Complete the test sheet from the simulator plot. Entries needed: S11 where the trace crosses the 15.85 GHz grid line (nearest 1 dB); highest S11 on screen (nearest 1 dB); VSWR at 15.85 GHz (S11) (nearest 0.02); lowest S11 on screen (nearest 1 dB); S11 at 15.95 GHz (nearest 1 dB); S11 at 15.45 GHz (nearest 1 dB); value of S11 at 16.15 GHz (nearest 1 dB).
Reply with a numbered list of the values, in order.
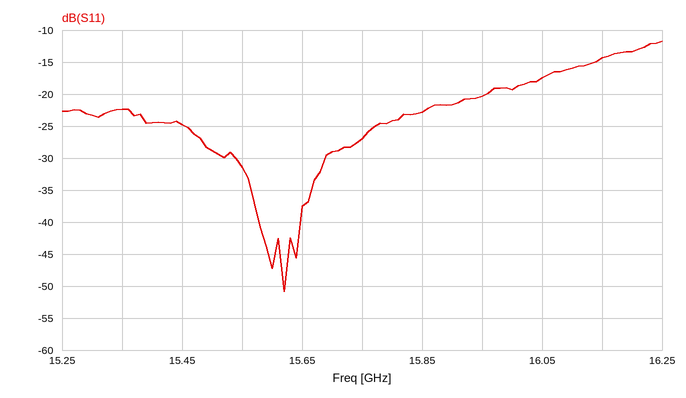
1. -23 dB
2. -12 dB
3. 1.16
4. -51 dB
5. -20 dB
6. -25 dB
7. -14 dB
